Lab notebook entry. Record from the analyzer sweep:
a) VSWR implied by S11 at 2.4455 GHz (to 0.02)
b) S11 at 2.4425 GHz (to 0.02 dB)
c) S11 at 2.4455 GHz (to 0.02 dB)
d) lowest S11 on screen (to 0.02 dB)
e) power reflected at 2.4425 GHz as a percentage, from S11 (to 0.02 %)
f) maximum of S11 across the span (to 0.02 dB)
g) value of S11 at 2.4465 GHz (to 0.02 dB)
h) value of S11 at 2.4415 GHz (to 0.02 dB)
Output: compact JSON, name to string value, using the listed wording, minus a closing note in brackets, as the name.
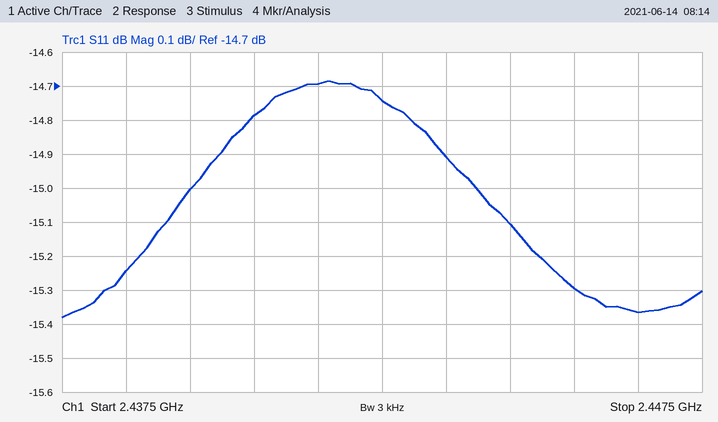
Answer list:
{"VSWR implied by S11 at 2.4455 GHz": "1.42", "S11 at 2.4425 GHz": "-14.74 dB", "S11 at 2.4455 GHz": "-15.30 dB", "lowest S11 on screen": "-15.38 dB", "power reflected at 2.4425 GHz as a percentage, from S11": "3.36 %", "maximum of S11 across the span": "-14.68 dB", "value of S11 at 2.4465 GHz": "-15.36 dB", "value of S11 at 2.4415 GHz": "-14.70 dB"}
